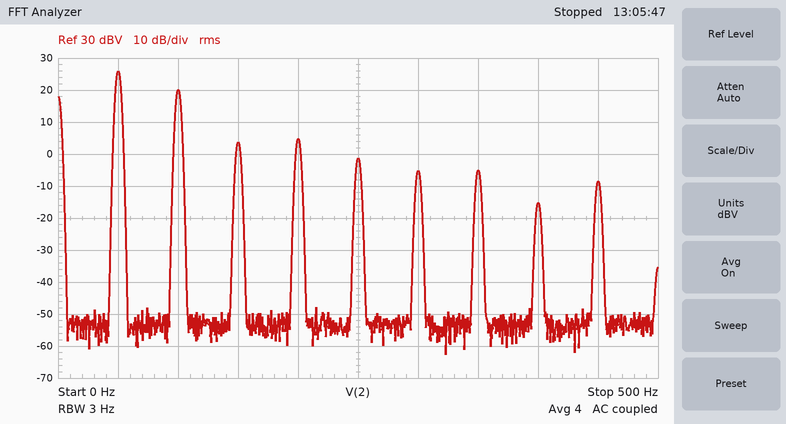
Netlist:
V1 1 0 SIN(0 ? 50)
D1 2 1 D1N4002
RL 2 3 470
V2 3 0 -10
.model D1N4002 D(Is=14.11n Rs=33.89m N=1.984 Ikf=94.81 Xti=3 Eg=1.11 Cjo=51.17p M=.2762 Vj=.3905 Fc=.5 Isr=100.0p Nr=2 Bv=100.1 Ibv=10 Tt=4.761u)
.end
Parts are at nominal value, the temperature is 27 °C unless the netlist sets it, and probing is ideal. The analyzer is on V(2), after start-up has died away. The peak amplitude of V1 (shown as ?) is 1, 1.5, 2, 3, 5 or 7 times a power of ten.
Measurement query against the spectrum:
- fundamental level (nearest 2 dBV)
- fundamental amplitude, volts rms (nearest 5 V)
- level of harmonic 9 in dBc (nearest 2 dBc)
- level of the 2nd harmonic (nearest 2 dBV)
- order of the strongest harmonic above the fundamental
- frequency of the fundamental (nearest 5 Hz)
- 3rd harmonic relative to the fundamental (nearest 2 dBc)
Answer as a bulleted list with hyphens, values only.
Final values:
- 26 dBV
- 20 V
- -34 dBc
- 20 dBV
- 2
- 50 Hz
- -22 dBc
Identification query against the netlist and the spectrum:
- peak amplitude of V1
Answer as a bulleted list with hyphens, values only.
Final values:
- 70 V
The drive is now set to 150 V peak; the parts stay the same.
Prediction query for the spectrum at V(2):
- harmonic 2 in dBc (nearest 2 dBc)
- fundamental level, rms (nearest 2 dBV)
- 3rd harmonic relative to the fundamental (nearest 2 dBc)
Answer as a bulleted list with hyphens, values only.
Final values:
- -16 dBc
- 36 dBV
- -18 dBc
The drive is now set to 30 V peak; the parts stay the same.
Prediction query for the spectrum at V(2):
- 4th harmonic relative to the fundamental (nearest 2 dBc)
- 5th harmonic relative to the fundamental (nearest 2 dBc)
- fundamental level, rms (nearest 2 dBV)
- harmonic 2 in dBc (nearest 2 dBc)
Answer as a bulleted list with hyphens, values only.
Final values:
- -30 dBc
- -22 dBc
- 16 dBV
- -4 dBc
